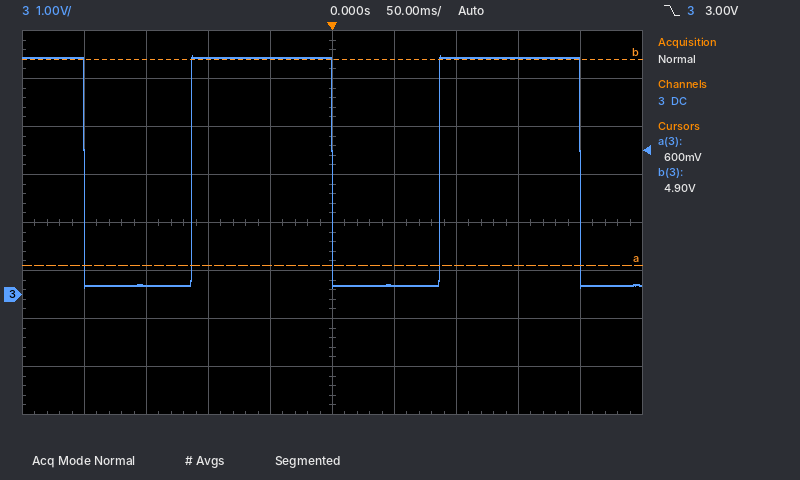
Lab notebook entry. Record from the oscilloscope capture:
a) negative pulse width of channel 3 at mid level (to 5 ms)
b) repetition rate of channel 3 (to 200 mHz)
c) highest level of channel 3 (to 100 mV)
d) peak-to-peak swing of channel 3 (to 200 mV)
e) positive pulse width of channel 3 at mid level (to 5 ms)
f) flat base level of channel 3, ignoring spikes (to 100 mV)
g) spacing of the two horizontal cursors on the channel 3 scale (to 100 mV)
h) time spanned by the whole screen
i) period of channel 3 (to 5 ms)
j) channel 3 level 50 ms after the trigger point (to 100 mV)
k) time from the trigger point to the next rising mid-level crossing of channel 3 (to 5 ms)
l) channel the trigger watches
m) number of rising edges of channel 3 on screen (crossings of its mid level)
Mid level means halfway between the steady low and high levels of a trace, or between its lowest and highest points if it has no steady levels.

85 ms
5.0 Hz
5.0 V
4.8 V
115 ms
200 mV
4.3 V
500 ms
200 ms
200 mV
85 ms
channel 3
2
